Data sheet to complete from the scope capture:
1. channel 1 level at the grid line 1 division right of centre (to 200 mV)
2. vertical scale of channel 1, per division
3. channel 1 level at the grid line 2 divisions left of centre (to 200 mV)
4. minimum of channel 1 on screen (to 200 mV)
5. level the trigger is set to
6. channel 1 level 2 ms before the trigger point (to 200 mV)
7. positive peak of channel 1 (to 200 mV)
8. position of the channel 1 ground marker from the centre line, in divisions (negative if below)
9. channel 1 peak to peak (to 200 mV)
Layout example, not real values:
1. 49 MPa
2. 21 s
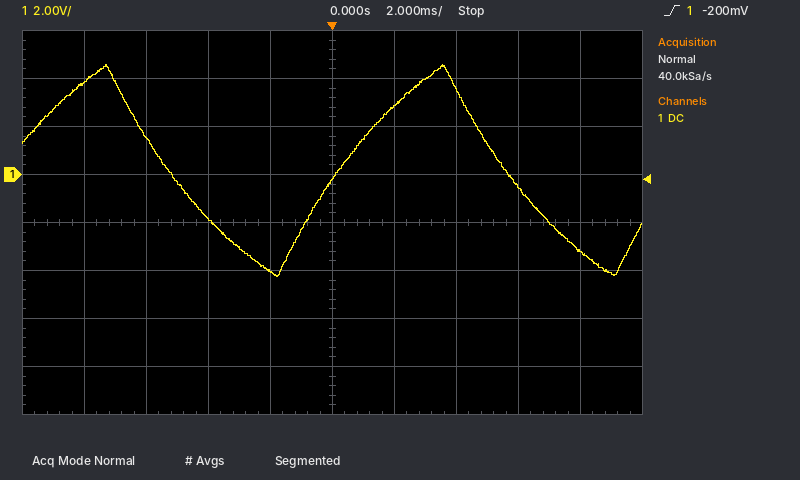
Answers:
1. 2.8 V
2. 2 V
3. -1.8 V
4. -4.2 V
5. -200 mV
6. -4.0 V
7. 4.6 V
8. +1.0 div
9. 8.8 V
